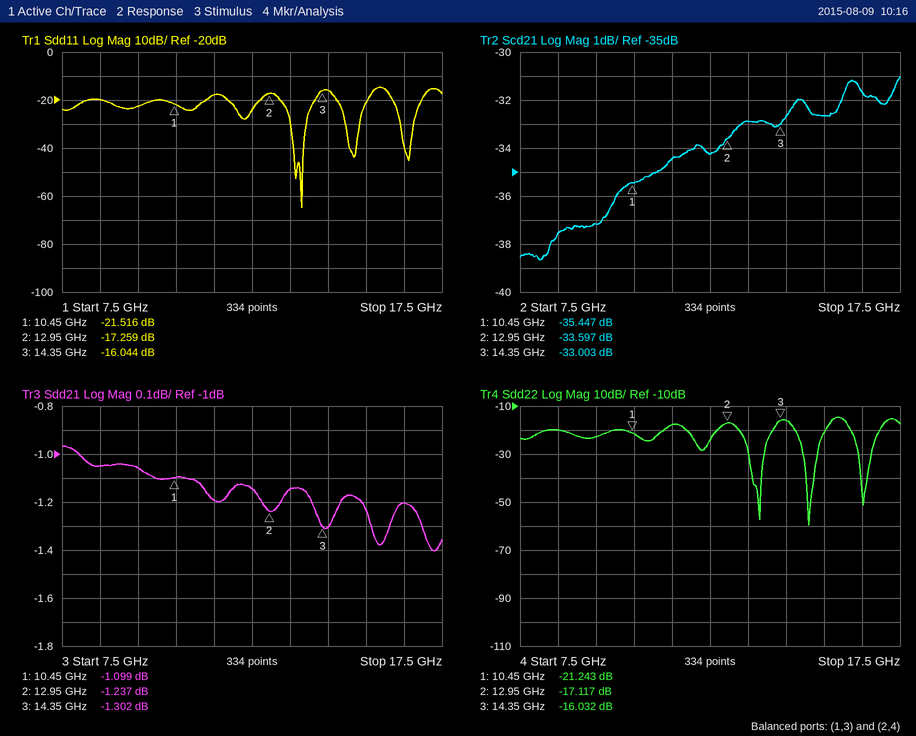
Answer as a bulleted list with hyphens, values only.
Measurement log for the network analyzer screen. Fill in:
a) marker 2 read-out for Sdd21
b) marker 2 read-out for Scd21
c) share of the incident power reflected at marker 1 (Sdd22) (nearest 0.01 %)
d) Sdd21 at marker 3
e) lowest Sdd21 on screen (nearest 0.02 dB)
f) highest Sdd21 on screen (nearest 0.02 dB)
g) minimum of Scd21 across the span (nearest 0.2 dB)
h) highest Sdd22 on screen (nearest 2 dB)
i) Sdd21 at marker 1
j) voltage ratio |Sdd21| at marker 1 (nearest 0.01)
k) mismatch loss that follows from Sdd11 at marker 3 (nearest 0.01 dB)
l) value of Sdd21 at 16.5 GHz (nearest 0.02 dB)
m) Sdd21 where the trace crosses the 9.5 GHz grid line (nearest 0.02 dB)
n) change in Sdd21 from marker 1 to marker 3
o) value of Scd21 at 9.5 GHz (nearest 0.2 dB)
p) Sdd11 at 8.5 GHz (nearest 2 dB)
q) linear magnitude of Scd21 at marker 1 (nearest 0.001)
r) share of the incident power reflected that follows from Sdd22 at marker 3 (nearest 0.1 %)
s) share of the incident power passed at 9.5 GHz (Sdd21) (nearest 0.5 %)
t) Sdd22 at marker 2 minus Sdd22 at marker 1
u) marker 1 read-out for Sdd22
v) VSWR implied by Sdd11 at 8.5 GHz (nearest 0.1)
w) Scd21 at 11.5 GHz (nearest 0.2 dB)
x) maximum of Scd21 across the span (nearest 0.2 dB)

- -1.237 dB
- -33.597 dB
- 0.75 %
- -1.302 dB
- -1.40 dB
- -0.96 dB
- -38.6 dB
- -14 dB
- -1.099 dB
- 0.88
- 0.11 dB
- -1.20 dB
- -1.06 dB
- -0.203 dB
- -37.2 dB
- -20 dB
- 0.017
- 2.5 %
- 78.5 %
- 4.126 dB
- -21.243 dB
- 1.2
- -34.4 dB
- -31.0 dB
